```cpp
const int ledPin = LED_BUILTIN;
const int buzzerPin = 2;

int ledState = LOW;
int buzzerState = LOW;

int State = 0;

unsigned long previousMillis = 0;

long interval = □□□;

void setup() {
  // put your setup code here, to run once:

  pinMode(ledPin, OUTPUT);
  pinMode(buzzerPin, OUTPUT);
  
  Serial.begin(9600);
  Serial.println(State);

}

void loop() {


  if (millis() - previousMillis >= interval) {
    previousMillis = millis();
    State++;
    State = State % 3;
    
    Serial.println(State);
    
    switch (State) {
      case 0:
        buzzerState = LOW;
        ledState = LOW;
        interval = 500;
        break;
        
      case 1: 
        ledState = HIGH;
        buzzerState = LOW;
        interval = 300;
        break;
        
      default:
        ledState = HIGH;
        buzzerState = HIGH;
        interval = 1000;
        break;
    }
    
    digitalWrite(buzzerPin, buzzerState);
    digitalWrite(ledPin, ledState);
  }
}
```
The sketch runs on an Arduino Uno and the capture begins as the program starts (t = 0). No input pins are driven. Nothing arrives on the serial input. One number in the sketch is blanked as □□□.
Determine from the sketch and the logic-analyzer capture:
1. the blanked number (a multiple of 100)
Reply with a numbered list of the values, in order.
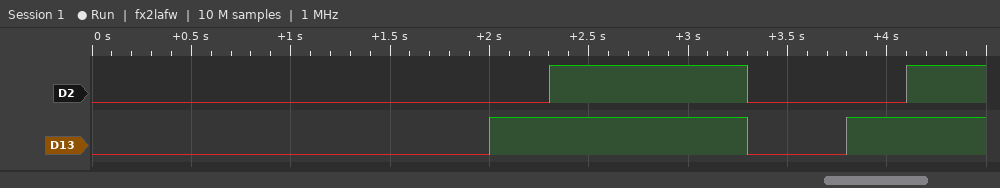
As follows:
1. 2000
